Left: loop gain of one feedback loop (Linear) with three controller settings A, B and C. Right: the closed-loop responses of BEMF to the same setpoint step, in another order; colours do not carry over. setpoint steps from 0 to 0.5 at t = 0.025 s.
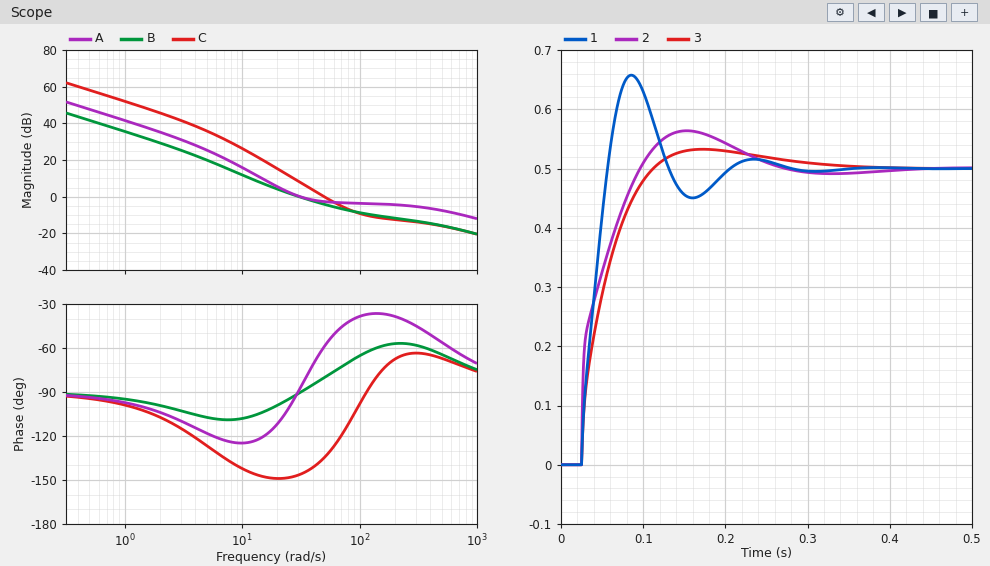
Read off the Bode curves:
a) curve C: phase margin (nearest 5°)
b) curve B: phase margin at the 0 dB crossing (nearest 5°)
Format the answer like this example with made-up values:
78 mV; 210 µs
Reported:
45°; 90°
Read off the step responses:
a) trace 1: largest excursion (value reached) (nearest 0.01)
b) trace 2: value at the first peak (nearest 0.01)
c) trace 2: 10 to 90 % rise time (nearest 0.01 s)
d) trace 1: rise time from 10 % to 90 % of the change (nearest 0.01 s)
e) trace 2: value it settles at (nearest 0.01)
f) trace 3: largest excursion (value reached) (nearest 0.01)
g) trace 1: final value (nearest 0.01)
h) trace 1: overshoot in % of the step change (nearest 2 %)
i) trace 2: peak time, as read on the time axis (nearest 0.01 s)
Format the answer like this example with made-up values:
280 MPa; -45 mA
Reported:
0.66; 0.56; 0.05 s; 0.03 s; 0.50; 0.53; 0.50; 32 %; 0.15 s
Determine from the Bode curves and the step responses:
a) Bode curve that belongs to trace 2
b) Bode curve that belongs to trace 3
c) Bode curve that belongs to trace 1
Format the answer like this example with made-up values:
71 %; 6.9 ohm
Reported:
A; B; C
